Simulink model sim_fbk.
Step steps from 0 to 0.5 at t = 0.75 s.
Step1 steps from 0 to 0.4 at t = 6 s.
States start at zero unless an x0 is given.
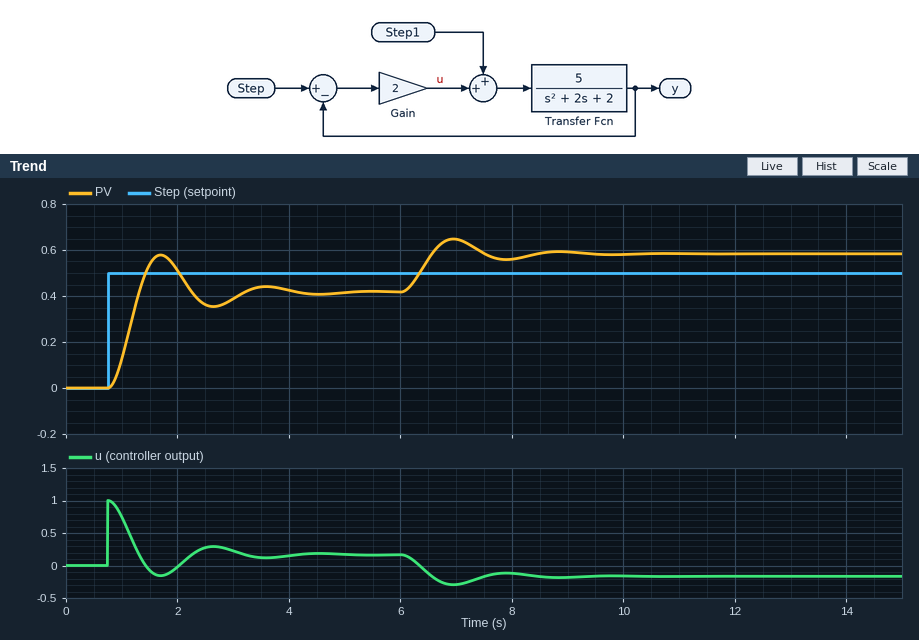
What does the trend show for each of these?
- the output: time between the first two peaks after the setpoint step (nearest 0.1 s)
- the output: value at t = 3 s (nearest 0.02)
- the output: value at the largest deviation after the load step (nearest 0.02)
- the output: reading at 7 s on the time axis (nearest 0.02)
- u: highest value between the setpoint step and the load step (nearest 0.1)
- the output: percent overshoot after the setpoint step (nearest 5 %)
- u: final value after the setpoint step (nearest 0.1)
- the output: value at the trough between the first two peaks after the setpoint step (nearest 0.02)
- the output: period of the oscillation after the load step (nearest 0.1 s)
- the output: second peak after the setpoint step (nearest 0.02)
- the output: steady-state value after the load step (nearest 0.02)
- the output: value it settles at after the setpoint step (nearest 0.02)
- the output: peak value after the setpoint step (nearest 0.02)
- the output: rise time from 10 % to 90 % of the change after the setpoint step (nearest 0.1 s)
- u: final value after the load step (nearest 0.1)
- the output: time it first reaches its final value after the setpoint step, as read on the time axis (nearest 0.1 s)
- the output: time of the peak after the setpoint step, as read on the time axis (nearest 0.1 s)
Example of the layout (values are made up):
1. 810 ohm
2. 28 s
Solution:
1. 1.9 s
2. 0.38
3. 0.64
4. 0.64
5. 1.0
6. 40 %
7. 0.2
8. 0.36
9. 1.9 s
10. 0.44
11. 0.58
12. 0.42
13. 0.58
14. 0.4 s
15. -0.2
16. 1.3 s
17. 1.7 s
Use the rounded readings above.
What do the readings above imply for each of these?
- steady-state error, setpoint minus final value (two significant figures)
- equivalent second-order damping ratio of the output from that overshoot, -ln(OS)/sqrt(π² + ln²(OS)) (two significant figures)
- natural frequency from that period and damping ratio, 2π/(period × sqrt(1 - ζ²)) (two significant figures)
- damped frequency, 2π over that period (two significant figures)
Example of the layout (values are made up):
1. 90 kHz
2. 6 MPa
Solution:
1. 0.080
2. 0.28
3. 3.4 rad/s
4. 3.3 rad/s
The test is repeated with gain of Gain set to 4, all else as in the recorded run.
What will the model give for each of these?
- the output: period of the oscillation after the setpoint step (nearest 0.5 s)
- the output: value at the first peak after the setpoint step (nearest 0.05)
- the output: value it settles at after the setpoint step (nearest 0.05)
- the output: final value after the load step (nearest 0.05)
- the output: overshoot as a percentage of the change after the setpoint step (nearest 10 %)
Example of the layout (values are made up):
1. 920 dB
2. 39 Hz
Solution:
1. 1.5 s
2. 0.70
3. 0.45
4. 0.55
5. 50 %
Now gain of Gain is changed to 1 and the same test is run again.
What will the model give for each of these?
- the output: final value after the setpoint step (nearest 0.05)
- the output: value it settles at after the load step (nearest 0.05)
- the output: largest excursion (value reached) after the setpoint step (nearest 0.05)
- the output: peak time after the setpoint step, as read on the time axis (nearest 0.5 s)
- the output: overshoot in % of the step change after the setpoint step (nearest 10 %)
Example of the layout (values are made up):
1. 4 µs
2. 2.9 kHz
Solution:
1. 0.35
2. 0.65
3. 0.45
4. 2.0 s
5. 30 %
